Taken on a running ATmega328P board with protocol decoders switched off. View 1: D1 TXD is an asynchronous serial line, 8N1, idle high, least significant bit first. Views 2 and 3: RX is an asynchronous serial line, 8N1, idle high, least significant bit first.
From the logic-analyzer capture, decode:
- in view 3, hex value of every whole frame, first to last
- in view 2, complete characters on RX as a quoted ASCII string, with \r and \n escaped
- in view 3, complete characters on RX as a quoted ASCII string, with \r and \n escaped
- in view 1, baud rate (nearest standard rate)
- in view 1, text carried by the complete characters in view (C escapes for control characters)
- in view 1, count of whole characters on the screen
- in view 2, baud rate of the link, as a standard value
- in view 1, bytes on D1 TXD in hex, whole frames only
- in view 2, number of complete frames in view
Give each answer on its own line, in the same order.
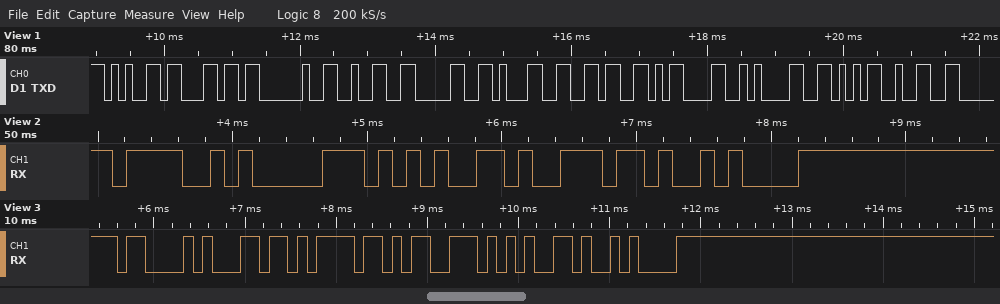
0x43 0x6C 0x6F 0x73 0x65 0x0A
"Open\n"
"Close\n"
9600 baud
"el 2016\r\nV2"
11
9600 baud
65 6C 20 32 30 31 36 0D 0A 56 32
5
